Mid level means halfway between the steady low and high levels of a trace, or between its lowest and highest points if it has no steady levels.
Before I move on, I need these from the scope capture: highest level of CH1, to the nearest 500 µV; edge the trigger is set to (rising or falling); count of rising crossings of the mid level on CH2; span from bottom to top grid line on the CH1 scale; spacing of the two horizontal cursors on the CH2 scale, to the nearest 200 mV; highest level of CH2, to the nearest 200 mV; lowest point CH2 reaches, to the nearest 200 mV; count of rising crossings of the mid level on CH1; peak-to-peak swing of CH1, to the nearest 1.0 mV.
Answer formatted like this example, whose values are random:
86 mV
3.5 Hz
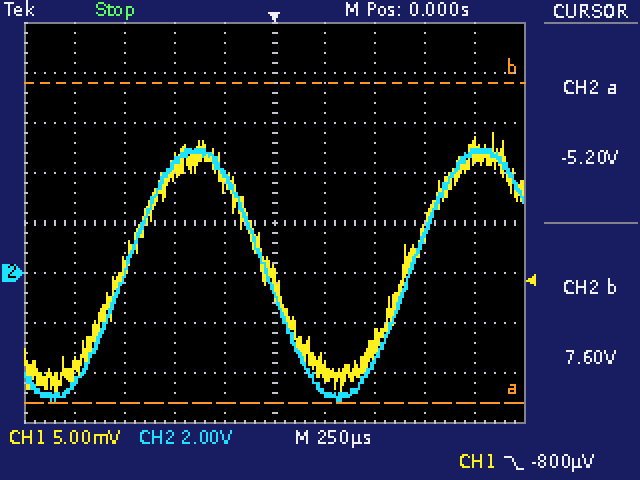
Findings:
14.0 mV
falling
2
40 mV
12.8 V
5.0 V
-5.2 V
2
26.0 mV
